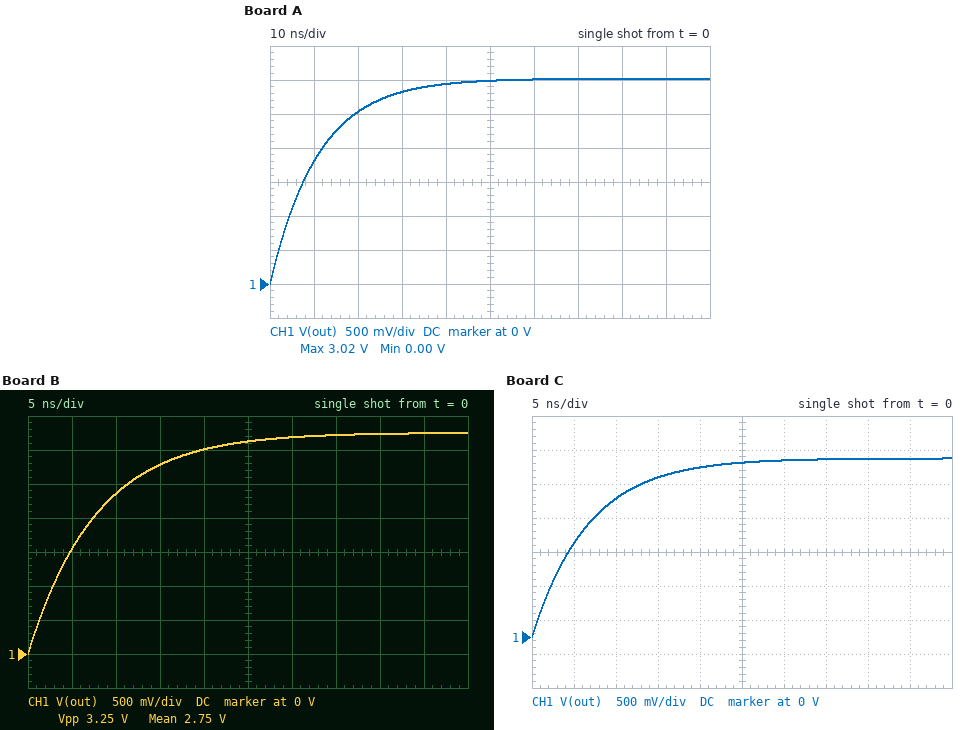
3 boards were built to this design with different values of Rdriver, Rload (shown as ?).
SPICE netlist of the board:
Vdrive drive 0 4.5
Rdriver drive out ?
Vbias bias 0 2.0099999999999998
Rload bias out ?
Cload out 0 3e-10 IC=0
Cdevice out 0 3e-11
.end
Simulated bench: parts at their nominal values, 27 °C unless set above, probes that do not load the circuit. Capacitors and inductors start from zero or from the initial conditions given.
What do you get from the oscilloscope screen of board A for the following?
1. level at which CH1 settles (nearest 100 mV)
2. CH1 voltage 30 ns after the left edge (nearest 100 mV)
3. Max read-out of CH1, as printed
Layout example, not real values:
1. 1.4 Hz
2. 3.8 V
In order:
1. 3.0 V
2. 2.8 V
3. 3.02 V
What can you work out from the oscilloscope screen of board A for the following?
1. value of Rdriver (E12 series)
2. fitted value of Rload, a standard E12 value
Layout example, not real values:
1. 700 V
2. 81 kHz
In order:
1. 82 Ω
2. 56 Ω
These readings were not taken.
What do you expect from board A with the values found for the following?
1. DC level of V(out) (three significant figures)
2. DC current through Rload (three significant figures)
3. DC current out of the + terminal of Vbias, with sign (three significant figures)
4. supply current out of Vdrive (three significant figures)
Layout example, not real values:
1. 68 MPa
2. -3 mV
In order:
1. 3.02 V
2. 18.0 mA
3. -18.0 mA
4. 18.0 mA
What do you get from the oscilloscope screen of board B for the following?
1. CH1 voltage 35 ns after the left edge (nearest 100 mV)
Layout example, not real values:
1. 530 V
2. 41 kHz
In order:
1. 3.2 V
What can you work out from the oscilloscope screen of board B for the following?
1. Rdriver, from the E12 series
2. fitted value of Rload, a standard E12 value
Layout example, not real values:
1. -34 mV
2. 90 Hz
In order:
1. 47 Ω
2. 47 Ω
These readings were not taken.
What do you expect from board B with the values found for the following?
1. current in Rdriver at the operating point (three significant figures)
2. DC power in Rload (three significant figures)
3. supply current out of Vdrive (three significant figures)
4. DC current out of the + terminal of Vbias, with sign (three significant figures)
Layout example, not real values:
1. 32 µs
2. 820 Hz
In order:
1. 26.5 mA
2. 33.0 mW
3. 26.5 mA
4. -26.5 mA
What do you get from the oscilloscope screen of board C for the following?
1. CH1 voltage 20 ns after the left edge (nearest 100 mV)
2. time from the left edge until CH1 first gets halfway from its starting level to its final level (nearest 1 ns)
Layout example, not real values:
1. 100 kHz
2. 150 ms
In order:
1. 2.5 V
2. 5 ns
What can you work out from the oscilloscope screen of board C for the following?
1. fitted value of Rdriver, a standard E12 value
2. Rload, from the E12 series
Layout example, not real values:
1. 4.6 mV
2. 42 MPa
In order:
1. 82 Ω
2. 27 Ω
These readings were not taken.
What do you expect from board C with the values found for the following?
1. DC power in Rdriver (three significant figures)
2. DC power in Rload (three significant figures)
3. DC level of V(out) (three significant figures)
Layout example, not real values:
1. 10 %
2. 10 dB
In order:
1. 42.8 mW
2. 14.1 mW
3. 2.63 V
